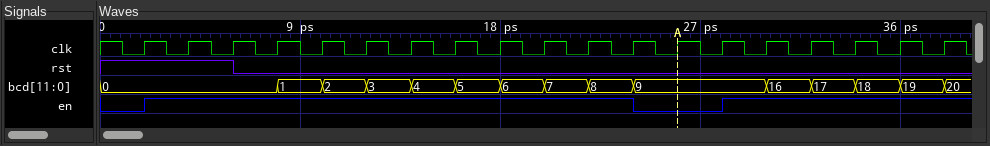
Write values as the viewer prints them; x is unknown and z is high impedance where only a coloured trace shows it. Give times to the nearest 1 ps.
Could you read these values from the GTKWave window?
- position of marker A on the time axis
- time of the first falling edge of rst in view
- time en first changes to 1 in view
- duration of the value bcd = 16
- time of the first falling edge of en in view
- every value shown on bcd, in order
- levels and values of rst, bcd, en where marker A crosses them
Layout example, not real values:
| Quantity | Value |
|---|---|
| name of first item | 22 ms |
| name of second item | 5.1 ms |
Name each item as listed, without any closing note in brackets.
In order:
| Quantity | Value |
|---|---|
| position of marker A on the time axis | 26 ps |
| time of the first falling edge of rst in view | 6 ps |
| time en first changes to 1 in view | 2 ps |
| duration of the value bcd = 16 | 2 ps |
| time of the first falling edge of en in view | 24 ps |
| every value shown on bcd, in order | 0, 1, 2, 3, 4, 5, 6, 7, 8, 9, 16, 17, 18, 19, 20 |
| levels and values of rst, bcd, en where marker A crosses them | rst=0, bcd=9, en=0 |
